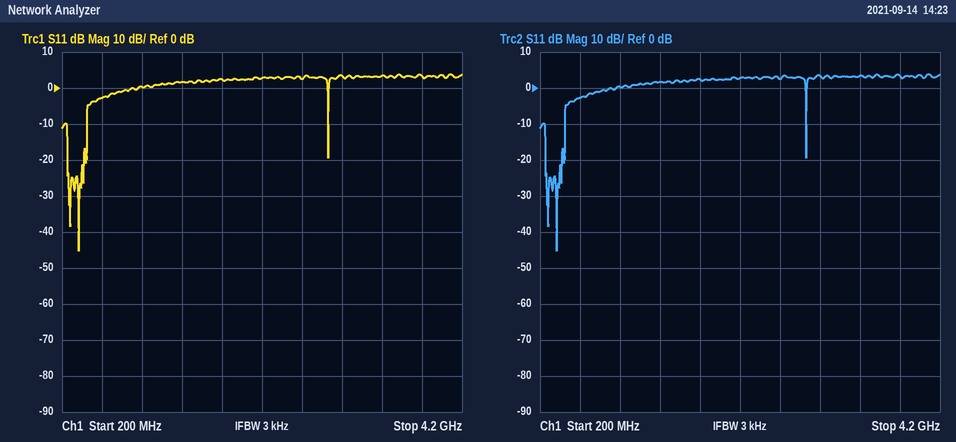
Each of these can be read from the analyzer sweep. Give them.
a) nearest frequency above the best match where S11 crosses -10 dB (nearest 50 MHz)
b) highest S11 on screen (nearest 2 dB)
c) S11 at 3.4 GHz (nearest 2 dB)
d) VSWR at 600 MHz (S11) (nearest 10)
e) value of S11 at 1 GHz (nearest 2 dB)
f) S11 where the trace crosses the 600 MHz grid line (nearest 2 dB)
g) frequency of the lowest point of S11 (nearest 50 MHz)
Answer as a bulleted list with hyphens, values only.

- 450 MHz
- 4 dB
- 4 dB
- 10
- 0 dB
- -2 dB
- 350 MHz
